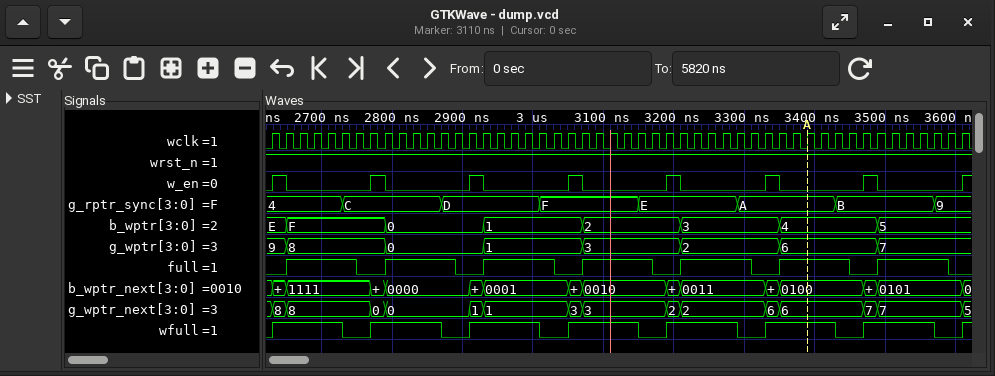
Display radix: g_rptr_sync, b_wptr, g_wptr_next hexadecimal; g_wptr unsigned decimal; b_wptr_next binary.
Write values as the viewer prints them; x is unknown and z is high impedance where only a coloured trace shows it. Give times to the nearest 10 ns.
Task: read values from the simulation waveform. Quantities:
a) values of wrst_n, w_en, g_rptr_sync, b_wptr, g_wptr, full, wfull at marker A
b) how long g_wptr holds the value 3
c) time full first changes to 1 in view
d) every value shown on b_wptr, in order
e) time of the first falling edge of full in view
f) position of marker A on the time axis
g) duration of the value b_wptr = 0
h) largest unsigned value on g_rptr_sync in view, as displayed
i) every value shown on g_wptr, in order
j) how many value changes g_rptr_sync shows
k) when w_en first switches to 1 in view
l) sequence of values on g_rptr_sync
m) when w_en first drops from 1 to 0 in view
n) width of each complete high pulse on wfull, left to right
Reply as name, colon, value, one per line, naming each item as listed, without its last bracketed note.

values of wrst_n, w_en, g_rptr_sync, b_wptr, g_wptr, full, wfull at marker A: wrst_n=1, w_en=0, g_rptr_sync=A, b_wptr=4, g_wptr=6, full=1, wfull=1
how long g_wptr holds the value 3: 140 ns
time full first changes to 1 in view: 2650 ns
every value shown on b_wptr, in order: E, F, 0, 1, 2, 3, 4, 5
time of the first falling edge of full in view: 2750 ns
position of marker A on the time axis: 3390 ns
duration of the value b_wptr = 0: 140 ns
largest unsigned value on g_rptr_sync in view, as displayed: F
every value shown on g_wptr, in order: 9, 8, 0, 1, 3, 2, 6, 7
how many value changes g_rptr_sync shows: 7
when w_en first switches to 1 in view: 2630 ns
sequence of values on g_rptr_sync: 4, C, D, F, E, A, B, 9
when w_en first drops from 1 to 0 in view: 2650 ns
width of each complete high pulse on wfull, left to right: 100 ns, 100 ns, 100 ns, 100 ns, 100 ns, 100 ns, 100 ns
